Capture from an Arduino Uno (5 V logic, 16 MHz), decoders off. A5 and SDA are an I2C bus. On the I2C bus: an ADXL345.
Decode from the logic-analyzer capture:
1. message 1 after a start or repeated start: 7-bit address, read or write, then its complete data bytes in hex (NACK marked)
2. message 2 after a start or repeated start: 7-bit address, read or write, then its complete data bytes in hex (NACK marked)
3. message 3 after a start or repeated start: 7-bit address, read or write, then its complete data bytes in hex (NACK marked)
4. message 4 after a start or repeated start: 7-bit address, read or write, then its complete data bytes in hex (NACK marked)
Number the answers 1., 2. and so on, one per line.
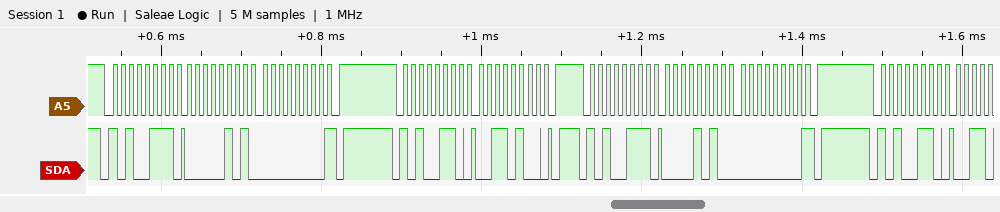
1. 0x53 read: 05 00 NACK
2. 0x53 write: 34
3. 0x53 read: 0A 00 NACK
4. 0x53 write
